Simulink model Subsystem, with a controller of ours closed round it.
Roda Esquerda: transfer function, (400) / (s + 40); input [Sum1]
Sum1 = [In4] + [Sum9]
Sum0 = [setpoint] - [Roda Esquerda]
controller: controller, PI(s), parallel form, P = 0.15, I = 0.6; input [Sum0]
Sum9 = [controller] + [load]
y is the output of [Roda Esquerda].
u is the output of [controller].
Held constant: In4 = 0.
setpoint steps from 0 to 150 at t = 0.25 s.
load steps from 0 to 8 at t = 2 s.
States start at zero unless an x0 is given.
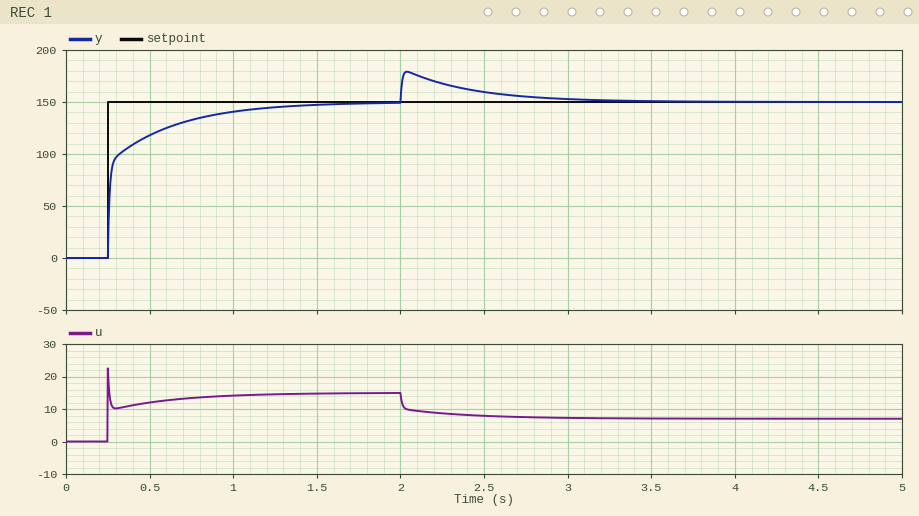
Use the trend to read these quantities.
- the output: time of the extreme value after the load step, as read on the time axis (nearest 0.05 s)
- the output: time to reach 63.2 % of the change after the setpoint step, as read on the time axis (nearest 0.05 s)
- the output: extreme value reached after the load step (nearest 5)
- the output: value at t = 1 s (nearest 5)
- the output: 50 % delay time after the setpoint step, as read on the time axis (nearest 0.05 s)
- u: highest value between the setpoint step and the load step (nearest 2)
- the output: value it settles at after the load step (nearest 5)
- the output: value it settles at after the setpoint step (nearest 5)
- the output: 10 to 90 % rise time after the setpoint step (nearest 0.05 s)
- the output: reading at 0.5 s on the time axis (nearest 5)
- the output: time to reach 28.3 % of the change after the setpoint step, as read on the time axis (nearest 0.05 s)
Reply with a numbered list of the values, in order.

1. 2.05 s
2. 0.30 s
3. 180
4. 140
5. 0.25 s
6. 22
7. 150
8. 150
9. 0.55 s
10. 120
11. 0.25 s
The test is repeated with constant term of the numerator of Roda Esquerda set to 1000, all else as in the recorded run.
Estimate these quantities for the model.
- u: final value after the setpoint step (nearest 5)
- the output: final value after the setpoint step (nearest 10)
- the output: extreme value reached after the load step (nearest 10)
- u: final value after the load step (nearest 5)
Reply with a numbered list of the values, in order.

1. 5
2. 150
3. 190
4. 0
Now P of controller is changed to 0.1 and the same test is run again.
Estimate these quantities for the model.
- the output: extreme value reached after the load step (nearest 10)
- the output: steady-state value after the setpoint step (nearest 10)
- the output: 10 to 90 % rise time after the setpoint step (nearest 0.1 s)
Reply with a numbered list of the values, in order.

1. 190
2. 150
3. 0.5 s
